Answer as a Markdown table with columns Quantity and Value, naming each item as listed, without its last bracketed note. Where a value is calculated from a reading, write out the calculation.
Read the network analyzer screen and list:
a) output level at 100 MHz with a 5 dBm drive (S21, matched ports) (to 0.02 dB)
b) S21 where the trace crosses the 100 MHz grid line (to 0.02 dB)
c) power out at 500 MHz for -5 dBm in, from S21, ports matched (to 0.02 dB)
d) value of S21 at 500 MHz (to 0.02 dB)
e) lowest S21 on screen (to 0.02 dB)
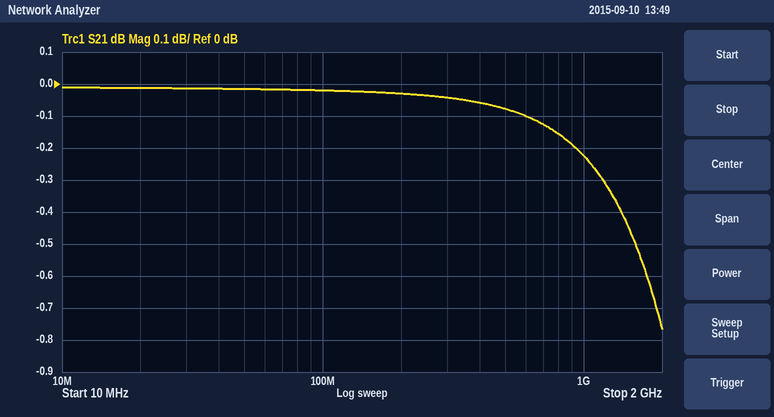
| Quantity | Value |
|---|---|
| output level at 100 MHz with a 5 dBm drive (S21, matched ports) | 5 dBm + (-0.02 dB) = 4.98 dBm |
| S21 where the trace crosses the 100 MHz grid line | -0.02 dB |
| power out at 500 MHz for -5 dBm in, from S21, ports matched | -5 dBm + (-0.08 dB) = -5.08 dBm |
| value of S21 at 500 MHz | -0.08 dB |
| lowest S21 on screen | -0.76 dB |
